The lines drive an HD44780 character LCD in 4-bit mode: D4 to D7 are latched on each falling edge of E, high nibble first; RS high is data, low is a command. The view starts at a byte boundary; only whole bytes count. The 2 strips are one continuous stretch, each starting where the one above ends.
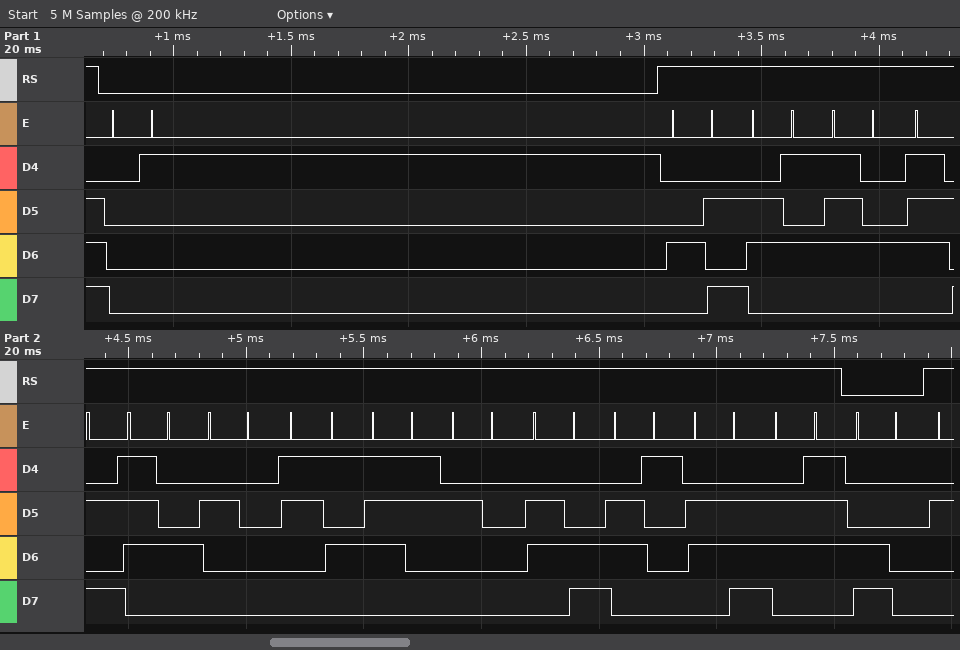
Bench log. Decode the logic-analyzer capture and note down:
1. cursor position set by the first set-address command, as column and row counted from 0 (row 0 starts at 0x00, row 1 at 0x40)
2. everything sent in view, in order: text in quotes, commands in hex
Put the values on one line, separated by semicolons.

column 0, row 1; 0x01 "Jetzt 5s lang" 0xC0
